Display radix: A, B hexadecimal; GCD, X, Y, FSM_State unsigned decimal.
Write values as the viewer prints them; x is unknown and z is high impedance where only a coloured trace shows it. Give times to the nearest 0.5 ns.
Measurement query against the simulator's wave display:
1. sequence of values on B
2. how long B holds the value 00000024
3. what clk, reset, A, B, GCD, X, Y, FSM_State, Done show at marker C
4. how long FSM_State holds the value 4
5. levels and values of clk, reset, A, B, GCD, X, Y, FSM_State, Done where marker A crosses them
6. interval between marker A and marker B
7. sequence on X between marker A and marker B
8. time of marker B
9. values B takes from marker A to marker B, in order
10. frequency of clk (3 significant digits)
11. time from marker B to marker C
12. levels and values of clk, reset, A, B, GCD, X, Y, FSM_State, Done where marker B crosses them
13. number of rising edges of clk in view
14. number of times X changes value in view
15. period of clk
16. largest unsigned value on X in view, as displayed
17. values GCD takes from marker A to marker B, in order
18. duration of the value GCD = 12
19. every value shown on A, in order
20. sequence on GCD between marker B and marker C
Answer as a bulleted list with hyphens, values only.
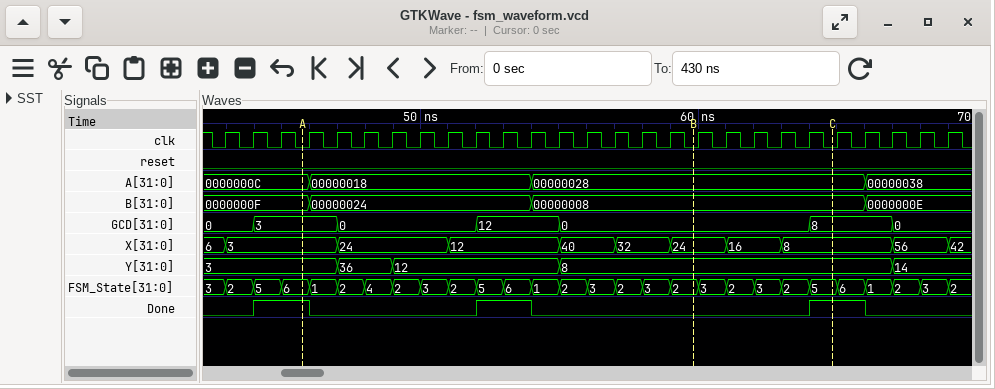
- 0000000F, 00000024, 00000008, 0000000E
- 8 ns
- clk=0, reset=0, A=00000028, B=00000008, GCD=8, X=8, Y=8, FSM_State=5, Done=1
- 1 ns
- clk=0, reset=0, A=0000000C, B=0000000F, GCD=3, X=3, Y=3, FSM_State=6, Done=1
- 14 ns
- 3, 24, 12, 40, 32, 24
- 60 ns
- 0000000F, 00000024, 00000008
- 1.00 GHz
- 5 ns
- clk=0, reset=0, A=00000028, B=00000008, GCD=0, X=24, Y=8, FSM_State=2, Done=0
- 27
- 10
- 1 ns
- 56
- 3, 0, 12, 0
- 3 ns
- 0000000C, 00000018, 00000028, 00000038
- 0, 8
